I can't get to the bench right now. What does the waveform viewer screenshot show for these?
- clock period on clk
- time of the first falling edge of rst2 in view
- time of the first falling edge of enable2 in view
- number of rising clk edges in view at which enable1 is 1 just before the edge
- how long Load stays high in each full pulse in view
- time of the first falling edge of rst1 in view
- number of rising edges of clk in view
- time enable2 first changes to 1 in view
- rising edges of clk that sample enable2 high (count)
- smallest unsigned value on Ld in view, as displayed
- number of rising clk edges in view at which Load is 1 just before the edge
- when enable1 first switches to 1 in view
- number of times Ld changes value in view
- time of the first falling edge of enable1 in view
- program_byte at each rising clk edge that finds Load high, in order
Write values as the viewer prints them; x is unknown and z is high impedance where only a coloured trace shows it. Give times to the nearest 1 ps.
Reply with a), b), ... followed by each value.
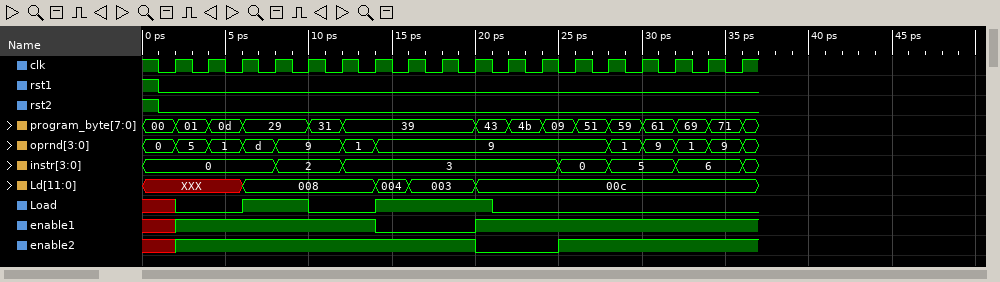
a) 2 ps
b) 1 ps
c) 20 ps
d) 14
e) 4 ps, 7 ps
f) 1 ps
g) 18
h) 2 ps
i) 15
j) 003
k) 5
l) 2 ps
m) 4
n) 14 ps
o) 29, 29, 39, 39, 39
